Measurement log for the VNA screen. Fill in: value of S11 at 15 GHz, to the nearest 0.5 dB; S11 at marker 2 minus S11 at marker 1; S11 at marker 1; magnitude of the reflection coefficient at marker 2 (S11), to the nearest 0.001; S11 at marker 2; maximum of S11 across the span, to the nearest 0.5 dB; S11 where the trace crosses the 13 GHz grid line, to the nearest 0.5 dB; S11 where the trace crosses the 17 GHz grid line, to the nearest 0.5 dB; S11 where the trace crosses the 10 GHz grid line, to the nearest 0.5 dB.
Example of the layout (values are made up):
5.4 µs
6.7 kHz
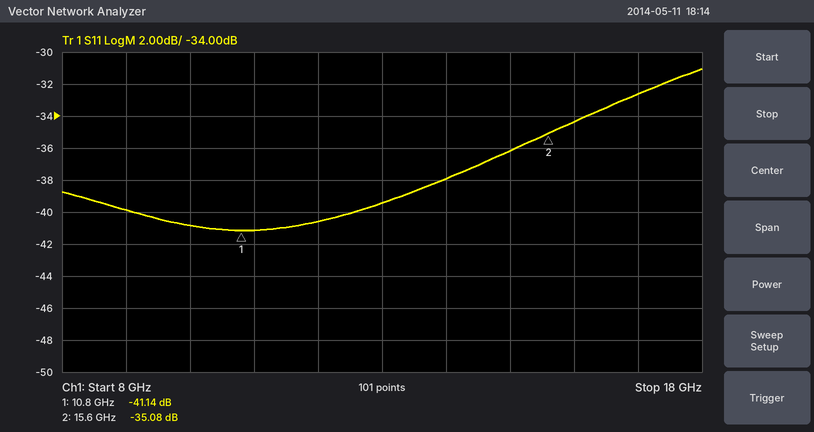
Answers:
-36.0 dB
6.06 dB
-41.14 dB
0.018
-35.08 dB
-31.0 dB
-39.5 dB
-32.5 dB
-41.0 dB
